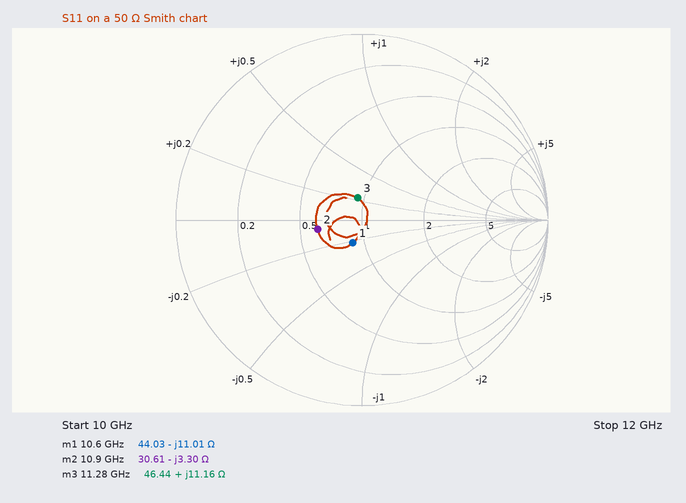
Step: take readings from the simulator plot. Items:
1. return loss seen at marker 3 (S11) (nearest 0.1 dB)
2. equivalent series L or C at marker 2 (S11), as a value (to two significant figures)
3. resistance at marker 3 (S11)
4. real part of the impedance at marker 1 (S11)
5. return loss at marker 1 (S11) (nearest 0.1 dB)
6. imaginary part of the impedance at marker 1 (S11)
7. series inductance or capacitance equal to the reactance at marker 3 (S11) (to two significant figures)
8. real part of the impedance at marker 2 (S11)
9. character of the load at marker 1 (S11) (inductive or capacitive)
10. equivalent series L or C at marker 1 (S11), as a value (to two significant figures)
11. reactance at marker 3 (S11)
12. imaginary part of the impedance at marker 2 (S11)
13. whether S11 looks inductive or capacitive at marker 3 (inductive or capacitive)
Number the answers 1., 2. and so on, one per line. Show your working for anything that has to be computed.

1. 18.4 dB
2. C = 1/(2π × 10.9 GHz × 3.3 Ω) ≈ 4.4 pF
3. 46.44 Ω
4. 44.03 Ω
5. 17.6 dB
6. -11.01 Ω
7. L = 11.16 Ω/(2π × 11.28 GHz) ≈ 157 pH, so 160 pH to two significant figures
8. 30.61 Ω
9. capacitive
10. C = 1/(2π × 10.6 GHz × 11.01 Ω) ≈ 1.4 pF
11. +11.16 Ω
12. -3.30 Ω
13. inductive
